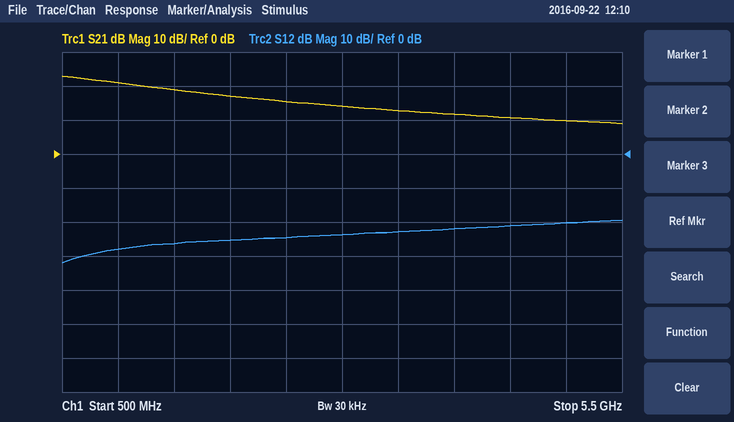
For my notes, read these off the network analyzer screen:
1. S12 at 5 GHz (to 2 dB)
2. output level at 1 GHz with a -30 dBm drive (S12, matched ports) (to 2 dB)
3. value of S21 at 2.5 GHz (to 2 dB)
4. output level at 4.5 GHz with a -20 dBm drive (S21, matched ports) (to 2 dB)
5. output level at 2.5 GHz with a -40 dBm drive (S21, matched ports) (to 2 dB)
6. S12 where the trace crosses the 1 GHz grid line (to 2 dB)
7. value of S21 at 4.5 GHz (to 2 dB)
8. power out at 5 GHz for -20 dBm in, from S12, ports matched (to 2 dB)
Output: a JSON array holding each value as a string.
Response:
["-20 dB", "-58 dBm", "16 dB", "-10 dBm", "-24 dBm", "-28 dB", "10 dB", "-40 dBm"]
